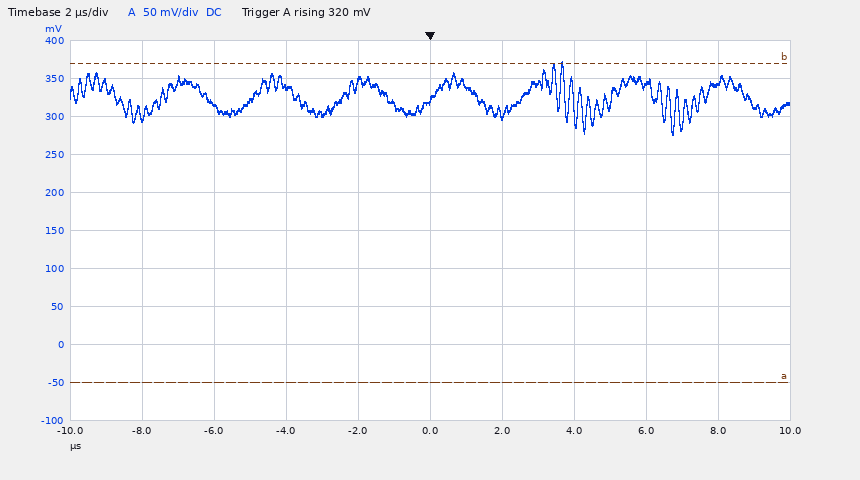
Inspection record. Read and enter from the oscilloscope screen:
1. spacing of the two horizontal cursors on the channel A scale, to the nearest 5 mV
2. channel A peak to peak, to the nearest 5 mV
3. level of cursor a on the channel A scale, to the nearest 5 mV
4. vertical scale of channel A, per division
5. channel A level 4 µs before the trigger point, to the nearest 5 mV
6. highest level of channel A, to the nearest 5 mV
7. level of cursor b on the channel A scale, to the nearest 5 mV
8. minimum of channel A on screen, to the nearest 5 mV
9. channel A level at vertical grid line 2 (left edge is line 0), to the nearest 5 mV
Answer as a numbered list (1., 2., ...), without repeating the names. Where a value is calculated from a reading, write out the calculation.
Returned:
1. 420 mV
2. 370 mV − (275 mV) = 95 mV
3. -50 mV
4. 50 mV
5. 340 mV
6. 370 mV
7. 370 mV
8. 275 mV
9. 315 mV
